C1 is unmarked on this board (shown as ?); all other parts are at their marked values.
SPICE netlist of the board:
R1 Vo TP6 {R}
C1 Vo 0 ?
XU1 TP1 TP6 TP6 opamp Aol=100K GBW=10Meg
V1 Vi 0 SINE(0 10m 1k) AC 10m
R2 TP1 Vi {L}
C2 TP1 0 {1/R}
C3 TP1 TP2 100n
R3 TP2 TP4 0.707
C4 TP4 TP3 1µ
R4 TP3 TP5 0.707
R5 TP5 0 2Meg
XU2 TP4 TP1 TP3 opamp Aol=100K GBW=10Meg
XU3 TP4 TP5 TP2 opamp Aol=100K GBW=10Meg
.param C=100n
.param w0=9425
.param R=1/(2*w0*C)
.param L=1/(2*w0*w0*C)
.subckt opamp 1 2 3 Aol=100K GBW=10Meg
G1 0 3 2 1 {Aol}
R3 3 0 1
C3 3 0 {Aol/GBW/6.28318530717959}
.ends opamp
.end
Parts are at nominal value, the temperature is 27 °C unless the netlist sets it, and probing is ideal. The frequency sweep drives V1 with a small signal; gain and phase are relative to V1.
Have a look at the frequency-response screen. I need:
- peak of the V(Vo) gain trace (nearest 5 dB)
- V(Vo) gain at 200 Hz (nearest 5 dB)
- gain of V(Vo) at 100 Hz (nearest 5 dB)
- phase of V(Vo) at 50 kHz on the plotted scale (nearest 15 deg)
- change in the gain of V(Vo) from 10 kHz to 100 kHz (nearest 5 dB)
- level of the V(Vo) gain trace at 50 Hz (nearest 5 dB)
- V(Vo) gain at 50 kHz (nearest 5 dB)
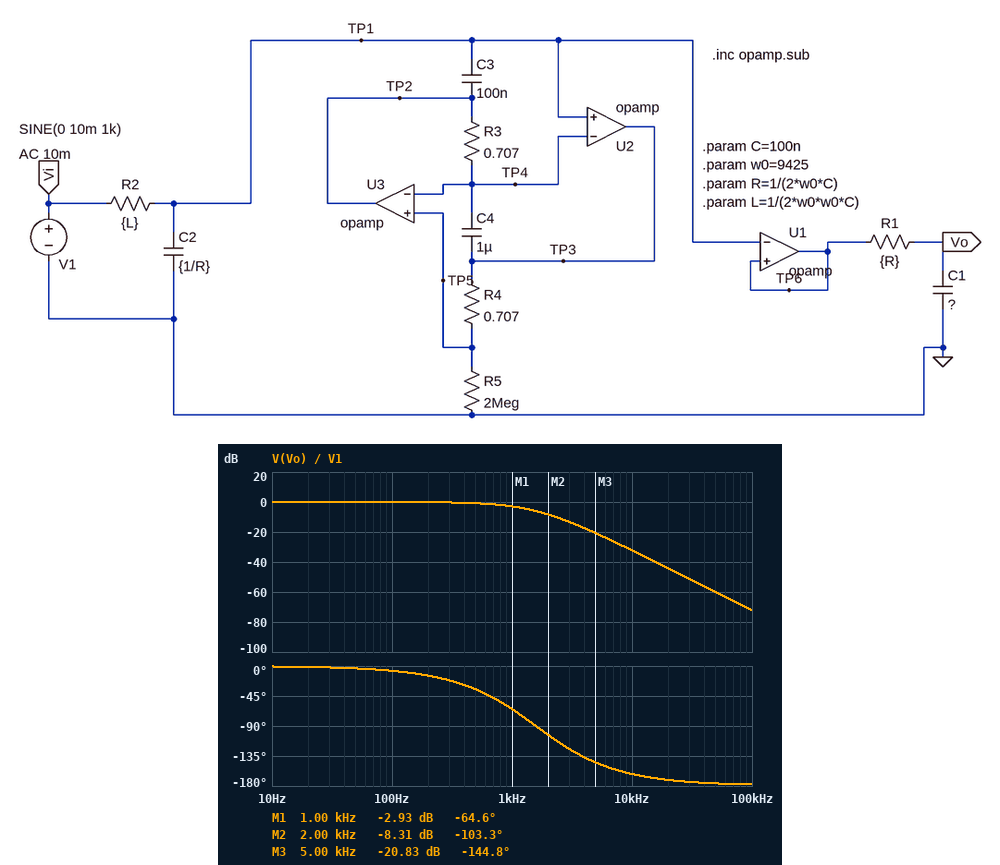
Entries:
0 dB
0 dB
0 dB
-180 deg
-40 dB
0 dB
-60 dB
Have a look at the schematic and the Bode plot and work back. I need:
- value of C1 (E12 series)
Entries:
180 nF
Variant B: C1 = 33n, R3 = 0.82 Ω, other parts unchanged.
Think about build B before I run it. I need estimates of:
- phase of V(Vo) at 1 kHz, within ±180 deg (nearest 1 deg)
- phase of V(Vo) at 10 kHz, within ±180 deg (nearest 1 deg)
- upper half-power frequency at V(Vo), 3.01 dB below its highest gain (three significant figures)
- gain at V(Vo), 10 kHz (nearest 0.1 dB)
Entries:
-40 deg
-129 deg
1.46 kHz
-20.0 dB
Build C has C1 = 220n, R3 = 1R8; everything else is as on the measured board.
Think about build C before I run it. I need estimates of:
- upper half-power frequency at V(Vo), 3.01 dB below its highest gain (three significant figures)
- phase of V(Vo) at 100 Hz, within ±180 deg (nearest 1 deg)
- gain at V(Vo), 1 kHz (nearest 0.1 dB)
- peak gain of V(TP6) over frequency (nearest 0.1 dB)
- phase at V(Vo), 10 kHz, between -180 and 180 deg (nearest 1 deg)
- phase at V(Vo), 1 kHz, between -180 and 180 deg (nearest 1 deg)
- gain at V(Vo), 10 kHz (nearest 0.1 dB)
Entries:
919 Hz
-8 deg
-3.5 dB
0 dB
-164 deg
-70 deg
-34.0 dB
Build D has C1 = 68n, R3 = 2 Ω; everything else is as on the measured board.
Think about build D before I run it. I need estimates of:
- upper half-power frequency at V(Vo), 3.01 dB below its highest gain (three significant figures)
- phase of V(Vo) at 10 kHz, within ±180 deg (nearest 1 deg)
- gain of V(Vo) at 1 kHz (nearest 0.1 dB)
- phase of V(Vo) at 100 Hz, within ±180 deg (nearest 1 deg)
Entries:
1.36 kHz
-148 deg
-1.8 dB
-5 deg
